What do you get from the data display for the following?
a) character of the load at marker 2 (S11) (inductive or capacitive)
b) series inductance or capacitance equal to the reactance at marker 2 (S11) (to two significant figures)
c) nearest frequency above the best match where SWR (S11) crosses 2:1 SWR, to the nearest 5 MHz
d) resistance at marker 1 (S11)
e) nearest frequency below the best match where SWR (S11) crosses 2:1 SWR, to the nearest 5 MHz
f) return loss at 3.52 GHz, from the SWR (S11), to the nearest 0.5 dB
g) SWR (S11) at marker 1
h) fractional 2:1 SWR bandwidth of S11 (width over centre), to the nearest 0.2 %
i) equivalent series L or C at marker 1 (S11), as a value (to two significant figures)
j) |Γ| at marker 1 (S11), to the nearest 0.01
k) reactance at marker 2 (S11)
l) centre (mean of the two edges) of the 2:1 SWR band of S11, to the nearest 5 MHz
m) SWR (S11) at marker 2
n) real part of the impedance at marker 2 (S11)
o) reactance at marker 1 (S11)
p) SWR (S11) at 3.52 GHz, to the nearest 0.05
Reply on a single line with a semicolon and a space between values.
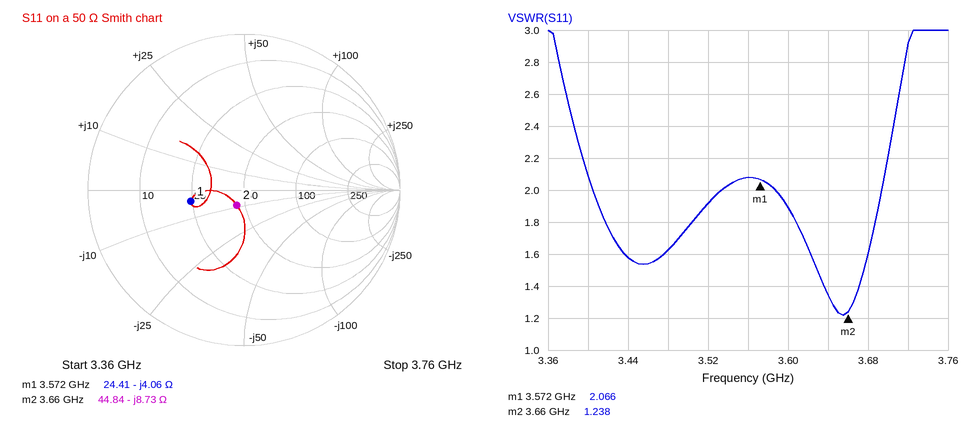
capacitive; 5.0 pF; 3.695 GHz; 24.41 Ω; 3.585 GHz; 10.0 dB; 2.066; 3.0 %; 11 pF; 0.35; -8.73 Ω; 3.640 GHz; 1.238; 44.84 Ω; -4.06 Ω; 1.90
